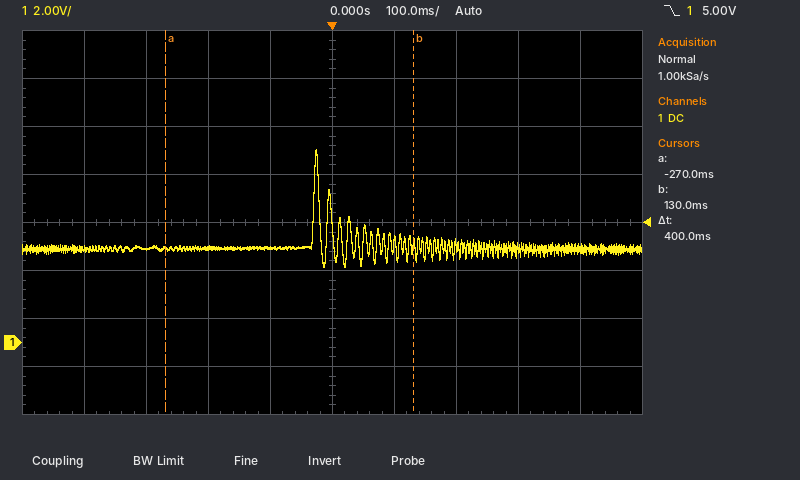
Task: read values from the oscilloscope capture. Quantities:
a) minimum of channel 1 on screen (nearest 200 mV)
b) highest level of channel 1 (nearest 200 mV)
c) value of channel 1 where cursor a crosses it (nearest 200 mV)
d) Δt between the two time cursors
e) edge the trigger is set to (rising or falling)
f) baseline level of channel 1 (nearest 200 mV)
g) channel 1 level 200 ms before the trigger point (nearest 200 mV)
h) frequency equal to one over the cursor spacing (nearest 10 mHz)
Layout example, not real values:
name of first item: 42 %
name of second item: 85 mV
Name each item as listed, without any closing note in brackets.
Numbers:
minimum of channel 1 on screen: 3.2 V
highest level of channel 1: 8.0 V
value of channel 1 where cursor a crosses it: 4.0 V
Δt between the two time cursors: 400 ms
edge the trigger is set to: falling
baseline level of channel 1: 4.0 V
channel 1 level 200 ms before the trigger point: 4.0 V
frequency equal to one over the cursor spacing: 2.50 Hz
